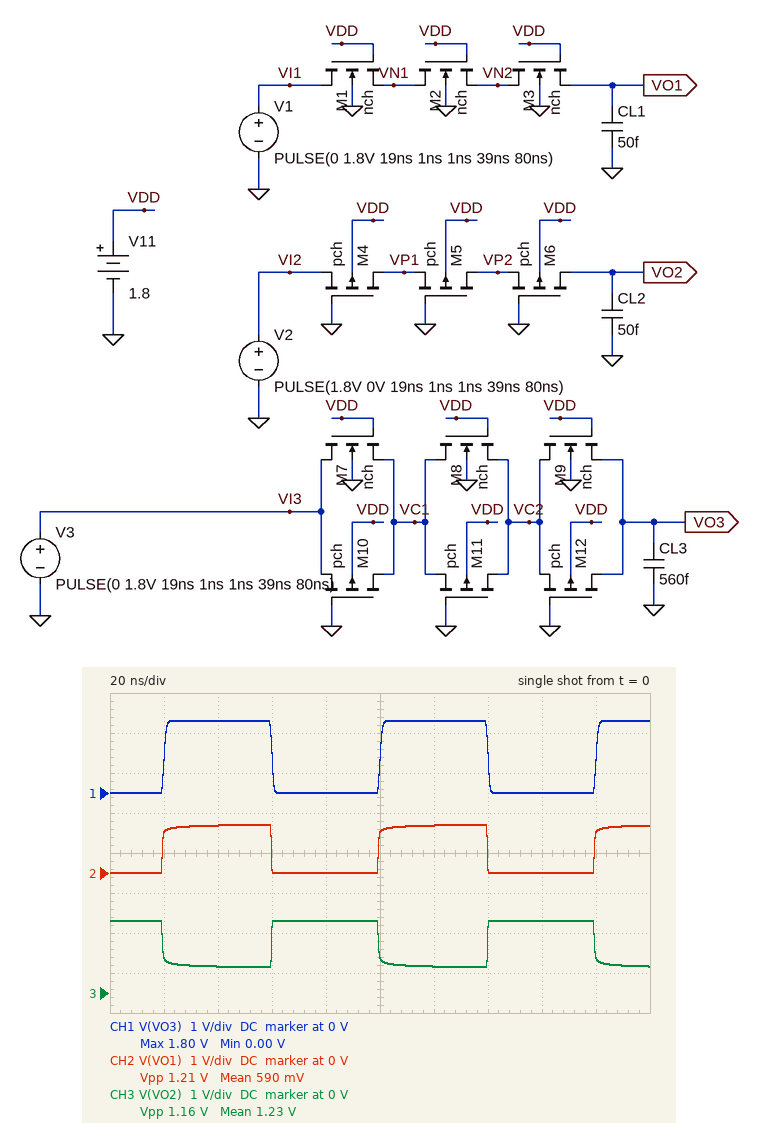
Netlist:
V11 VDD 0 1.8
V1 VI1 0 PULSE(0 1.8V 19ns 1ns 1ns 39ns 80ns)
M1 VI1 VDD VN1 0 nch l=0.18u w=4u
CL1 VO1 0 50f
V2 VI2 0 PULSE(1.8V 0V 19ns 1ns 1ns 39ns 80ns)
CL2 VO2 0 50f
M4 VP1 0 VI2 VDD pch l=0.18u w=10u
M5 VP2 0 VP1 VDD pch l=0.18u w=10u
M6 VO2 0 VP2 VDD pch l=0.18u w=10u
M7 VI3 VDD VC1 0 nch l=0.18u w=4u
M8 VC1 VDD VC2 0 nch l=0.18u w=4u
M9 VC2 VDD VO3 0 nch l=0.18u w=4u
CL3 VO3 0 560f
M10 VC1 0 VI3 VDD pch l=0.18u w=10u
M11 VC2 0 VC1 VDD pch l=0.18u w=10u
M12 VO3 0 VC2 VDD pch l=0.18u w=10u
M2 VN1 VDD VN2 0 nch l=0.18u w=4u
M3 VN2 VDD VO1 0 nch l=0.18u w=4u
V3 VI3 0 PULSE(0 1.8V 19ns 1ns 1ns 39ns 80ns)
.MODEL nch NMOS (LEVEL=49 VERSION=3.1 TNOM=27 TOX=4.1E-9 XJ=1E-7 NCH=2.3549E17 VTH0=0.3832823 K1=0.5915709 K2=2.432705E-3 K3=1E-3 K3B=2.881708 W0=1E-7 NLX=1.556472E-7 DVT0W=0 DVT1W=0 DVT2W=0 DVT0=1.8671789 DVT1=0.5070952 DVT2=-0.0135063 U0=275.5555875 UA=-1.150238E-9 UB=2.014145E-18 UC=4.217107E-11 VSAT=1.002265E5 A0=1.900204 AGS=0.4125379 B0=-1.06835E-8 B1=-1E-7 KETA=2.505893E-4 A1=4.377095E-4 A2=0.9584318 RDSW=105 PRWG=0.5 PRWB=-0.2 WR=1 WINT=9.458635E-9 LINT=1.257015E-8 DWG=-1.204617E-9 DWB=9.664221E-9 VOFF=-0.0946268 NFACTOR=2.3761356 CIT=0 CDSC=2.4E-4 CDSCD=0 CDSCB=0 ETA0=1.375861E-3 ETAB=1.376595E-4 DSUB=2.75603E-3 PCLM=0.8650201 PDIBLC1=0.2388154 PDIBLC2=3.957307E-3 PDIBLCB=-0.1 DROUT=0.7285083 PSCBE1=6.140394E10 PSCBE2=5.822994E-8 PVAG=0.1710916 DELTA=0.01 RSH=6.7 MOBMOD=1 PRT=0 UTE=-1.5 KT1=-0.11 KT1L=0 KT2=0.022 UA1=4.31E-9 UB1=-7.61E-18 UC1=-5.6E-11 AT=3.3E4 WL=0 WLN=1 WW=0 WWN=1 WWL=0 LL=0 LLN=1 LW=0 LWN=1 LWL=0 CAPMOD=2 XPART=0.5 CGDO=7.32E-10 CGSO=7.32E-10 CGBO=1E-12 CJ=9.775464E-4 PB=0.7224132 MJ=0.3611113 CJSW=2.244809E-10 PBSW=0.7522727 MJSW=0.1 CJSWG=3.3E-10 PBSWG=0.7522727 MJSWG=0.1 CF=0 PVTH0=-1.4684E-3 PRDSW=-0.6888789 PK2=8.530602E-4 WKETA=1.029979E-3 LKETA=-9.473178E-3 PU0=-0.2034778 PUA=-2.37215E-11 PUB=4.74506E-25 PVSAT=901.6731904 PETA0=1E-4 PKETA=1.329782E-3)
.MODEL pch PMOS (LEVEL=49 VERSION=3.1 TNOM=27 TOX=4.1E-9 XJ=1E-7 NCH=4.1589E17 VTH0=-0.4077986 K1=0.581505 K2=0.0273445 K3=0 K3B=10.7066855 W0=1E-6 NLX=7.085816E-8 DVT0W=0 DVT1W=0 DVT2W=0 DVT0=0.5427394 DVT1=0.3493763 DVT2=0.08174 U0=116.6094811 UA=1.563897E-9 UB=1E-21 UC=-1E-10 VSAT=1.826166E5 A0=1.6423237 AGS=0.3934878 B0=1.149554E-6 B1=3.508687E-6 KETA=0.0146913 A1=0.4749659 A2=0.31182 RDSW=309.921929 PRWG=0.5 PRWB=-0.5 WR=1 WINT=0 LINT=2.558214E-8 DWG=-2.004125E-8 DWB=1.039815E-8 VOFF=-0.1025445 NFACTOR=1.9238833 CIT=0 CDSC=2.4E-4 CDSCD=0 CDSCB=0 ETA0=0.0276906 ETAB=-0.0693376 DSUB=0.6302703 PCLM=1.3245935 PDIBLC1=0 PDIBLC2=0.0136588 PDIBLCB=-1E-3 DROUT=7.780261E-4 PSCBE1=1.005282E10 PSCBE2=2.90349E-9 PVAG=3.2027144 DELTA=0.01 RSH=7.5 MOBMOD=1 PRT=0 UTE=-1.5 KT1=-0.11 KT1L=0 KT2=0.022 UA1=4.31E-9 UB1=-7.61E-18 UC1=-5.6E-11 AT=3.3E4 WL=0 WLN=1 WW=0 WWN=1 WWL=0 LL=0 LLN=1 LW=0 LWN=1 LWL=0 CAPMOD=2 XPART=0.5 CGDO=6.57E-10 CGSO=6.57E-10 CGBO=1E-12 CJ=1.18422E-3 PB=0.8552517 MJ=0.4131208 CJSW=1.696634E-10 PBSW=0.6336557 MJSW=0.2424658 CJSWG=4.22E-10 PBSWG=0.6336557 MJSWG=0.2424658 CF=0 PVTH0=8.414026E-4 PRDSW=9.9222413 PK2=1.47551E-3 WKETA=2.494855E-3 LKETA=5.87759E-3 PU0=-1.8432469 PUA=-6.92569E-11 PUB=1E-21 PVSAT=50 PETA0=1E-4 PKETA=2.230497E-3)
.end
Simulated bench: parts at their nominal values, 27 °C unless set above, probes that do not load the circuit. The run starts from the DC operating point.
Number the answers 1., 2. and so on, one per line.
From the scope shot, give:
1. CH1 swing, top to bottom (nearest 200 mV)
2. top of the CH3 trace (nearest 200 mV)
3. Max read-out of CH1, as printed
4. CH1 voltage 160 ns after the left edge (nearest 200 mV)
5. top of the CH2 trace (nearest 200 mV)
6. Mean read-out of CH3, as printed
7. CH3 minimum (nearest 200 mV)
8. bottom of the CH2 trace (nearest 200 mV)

1. 1.8 V
2. 1.8 V
3. 1.80 V
4. 0 V
5. 1.2 V
6. 1.23 V
7. 600 mV
8. 0 V
